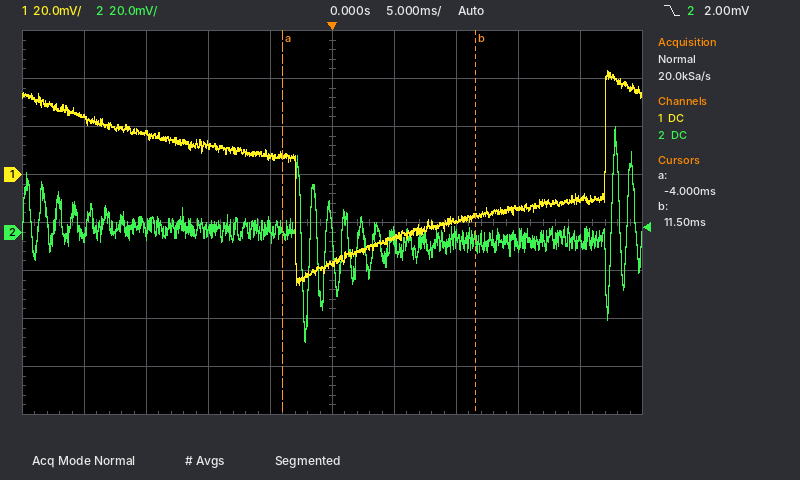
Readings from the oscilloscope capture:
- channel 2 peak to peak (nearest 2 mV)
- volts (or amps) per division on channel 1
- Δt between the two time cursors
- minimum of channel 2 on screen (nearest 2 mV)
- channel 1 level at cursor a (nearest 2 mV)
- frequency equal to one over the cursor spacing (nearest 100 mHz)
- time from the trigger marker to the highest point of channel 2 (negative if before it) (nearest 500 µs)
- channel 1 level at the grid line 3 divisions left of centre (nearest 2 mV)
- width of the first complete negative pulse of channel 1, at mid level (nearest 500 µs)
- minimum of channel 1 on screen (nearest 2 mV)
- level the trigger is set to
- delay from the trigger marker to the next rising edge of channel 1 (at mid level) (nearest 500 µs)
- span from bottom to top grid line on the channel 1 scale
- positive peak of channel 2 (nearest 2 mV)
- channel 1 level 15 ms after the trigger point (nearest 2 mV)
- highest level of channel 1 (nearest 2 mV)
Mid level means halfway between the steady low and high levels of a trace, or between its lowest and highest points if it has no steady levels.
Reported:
90 mV
20 mV
15.5 ms
-46 mV
8 mV
64.5 Hz
+23.0 ms
16 mV
25.0 ms
-46 mV
2.00 mV
22.0 ms
160 mV
44 mV
-14 mV
44 mV
